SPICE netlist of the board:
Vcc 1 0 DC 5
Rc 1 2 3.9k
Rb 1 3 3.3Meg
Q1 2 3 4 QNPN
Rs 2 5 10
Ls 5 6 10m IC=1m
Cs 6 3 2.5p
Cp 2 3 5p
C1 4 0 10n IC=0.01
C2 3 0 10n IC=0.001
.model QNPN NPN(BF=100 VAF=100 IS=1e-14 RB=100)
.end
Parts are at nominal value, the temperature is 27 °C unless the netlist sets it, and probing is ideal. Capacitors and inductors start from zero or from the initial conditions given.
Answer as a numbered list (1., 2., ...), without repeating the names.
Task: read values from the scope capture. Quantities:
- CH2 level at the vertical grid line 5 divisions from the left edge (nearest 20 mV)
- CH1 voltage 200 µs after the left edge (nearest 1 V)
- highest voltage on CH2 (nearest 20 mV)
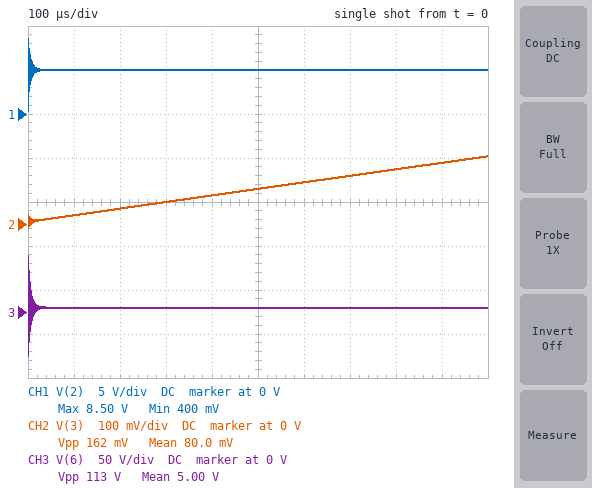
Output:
1. 80 mV
2. 5 V
3. 160 mV
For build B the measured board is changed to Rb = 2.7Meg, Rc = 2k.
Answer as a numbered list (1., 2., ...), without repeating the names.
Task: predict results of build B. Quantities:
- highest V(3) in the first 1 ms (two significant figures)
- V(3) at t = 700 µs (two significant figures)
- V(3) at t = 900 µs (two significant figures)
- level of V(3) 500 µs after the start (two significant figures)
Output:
1. 190 mV
2. 130 mV
3. 170 mV
4. 96 mV
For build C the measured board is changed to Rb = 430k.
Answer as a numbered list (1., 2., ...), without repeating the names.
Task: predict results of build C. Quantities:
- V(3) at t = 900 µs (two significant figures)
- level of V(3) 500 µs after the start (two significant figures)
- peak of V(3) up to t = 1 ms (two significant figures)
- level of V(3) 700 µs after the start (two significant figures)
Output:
1. 940 mV
2. 550 mV
3. 1.0 V
4. 750 mV
